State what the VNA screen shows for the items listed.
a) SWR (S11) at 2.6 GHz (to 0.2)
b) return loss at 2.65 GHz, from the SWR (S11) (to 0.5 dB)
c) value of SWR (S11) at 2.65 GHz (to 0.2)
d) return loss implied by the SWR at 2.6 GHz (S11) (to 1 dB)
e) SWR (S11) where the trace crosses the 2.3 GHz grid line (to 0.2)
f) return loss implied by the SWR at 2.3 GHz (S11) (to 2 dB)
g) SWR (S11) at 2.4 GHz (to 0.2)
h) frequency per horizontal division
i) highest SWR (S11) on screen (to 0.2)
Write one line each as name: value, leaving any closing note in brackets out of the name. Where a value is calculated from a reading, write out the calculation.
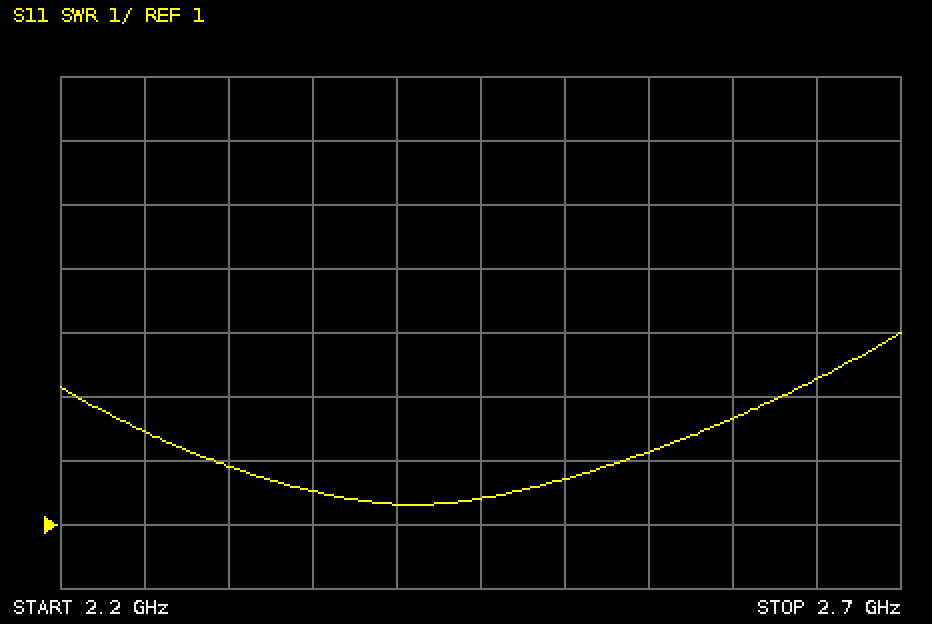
SWR (S11) at 2.6 GHz: 2.6
return loss at 2.65 GHz, from the SWR (S11): −20 log10((3.2 − 1)/(3.2 + 1)) ≈ 5.62 dB, so 5.5 dB to the nearest 0.5 dB
value of SWR (S11) at 2.65 GHz: 3.2
return loss implied by the SWR at 2.6 GHz (S11): −20 log10((2.6 − 1)/(2.6 + 1)) ≈ 7 dB
SWR (S11) where the trace crosses the 2.3 GHz grid line: 2.0
return loss implied by the SWR at 2.3 GHz (S11): −20 log10((2 − 1)/(2 + 1)) ≈ 10 dB
SWR (S11) at 2.4 GHz: 1.4
frequency per horizontal division: 50 MHz
highest SWR (S11) on screen: 4.0
